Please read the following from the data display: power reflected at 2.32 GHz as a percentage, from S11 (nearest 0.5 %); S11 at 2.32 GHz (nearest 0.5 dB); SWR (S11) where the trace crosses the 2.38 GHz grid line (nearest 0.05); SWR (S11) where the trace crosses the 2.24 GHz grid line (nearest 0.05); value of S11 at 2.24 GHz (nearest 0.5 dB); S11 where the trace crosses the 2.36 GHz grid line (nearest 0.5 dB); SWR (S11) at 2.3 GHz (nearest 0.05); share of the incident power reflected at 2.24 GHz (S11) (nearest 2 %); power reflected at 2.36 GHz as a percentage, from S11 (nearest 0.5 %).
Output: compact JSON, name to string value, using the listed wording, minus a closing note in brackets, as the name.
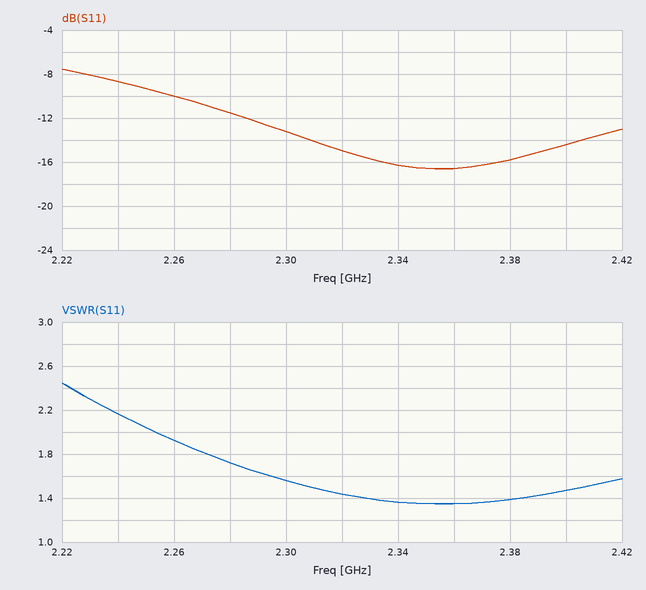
{"power reflected at 2.32 GHz as a percentage, from S11": "3.0 %", "S11 at 2.32 GHz": "-15.0 dB", "SWR (S11) where the trace crosses the 2.38 GHz grid line": "1.40", "SWR (S11) where the trace crosses the 2.24 GHz grid line": "2.15", "value of S11 at 2.24 GHz": "-8.5 dB", "S11 where the trace crosses the 2.36 GHz grid line": "-16.5 dB", "SWR (S11) at 2.3 GHz": "1.55", "share of the incident power reflected at 2.24 GHz (S11)": "14 %", "power reflected at 2.36 GHz as a percentage, from S11": "2.0 %"}
